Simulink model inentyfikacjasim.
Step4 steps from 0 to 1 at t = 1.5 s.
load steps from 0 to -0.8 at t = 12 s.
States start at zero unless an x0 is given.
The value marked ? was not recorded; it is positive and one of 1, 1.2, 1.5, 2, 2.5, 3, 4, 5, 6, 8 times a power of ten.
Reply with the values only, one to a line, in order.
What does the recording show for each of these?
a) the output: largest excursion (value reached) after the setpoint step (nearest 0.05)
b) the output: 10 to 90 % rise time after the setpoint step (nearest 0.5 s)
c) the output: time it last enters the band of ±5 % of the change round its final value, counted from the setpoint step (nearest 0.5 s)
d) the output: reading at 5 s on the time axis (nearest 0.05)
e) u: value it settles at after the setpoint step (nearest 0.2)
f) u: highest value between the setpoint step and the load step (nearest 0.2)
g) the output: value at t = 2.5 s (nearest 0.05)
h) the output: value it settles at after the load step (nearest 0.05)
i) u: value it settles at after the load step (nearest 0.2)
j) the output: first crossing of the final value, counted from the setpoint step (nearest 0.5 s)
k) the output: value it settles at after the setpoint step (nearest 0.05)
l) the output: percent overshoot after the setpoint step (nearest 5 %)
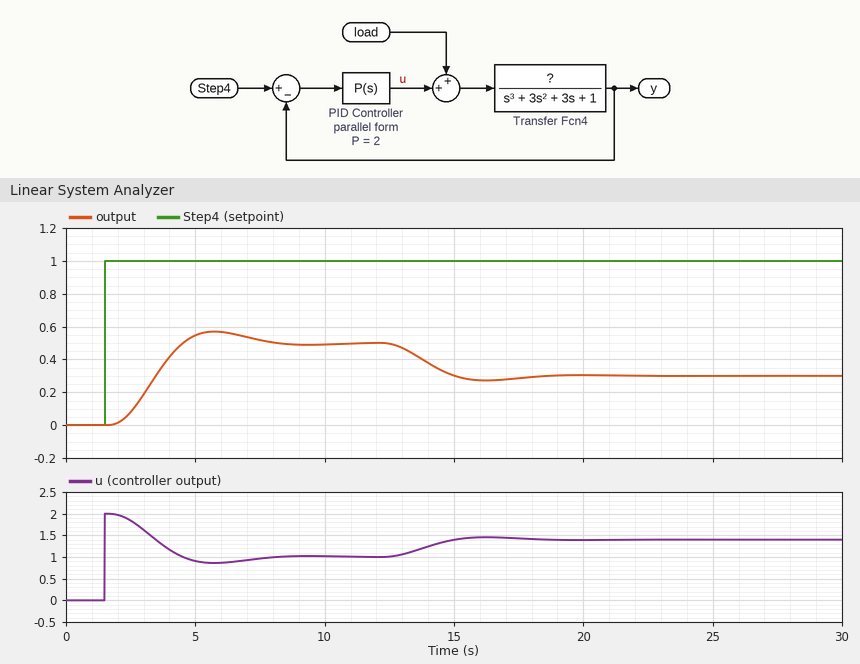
0.55
2.0 s
6.0 s
0.55
1.0
2.0
0.10
0.30
1.4
3.0 s
0.50
15 %
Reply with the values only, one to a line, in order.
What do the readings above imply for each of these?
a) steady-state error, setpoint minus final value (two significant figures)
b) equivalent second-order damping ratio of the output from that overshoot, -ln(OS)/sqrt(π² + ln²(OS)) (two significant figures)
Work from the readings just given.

0.50
0.52
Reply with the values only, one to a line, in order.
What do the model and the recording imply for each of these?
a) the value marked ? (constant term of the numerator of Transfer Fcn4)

0.5
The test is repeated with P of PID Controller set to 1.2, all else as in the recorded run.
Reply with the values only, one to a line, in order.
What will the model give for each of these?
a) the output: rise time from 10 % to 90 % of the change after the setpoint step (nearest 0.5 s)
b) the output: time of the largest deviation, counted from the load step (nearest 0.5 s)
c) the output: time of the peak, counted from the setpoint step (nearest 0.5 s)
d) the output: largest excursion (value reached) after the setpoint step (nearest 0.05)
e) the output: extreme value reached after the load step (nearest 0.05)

2.5 s
5.0 s
5.0 s
0.40
0.10
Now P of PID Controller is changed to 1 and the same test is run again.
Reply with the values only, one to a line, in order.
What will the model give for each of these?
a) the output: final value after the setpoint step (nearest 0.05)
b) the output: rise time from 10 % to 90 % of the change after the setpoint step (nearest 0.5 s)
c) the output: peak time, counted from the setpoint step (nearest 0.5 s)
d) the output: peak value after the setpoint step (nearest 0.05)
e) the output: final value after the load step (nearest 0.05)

0.35
2.5 s
5.5 s
0.35
0.05
